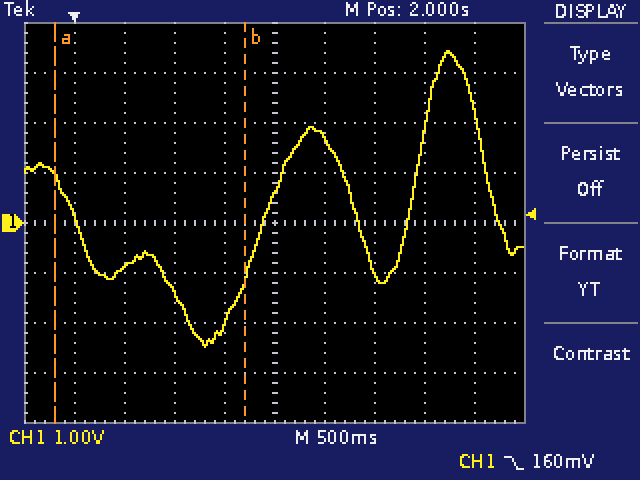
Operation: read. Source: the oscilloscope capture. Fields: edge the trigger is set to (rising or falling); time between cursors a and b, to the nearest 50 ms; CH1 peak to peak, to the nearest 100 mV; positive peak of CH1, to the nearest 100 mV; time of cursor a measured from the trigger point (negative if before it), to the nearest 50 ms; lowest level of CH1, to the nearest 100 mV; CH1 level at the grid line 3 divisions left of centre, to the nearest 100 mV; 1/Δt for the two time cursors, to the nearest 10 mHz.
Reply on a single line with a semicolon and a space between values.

falling; 1.90 s; 5.9 V; 3.4 V; -200 ms; -2.5 V; -900 mV; 530 mHz
